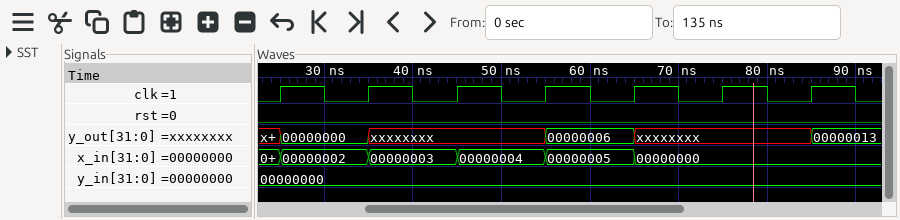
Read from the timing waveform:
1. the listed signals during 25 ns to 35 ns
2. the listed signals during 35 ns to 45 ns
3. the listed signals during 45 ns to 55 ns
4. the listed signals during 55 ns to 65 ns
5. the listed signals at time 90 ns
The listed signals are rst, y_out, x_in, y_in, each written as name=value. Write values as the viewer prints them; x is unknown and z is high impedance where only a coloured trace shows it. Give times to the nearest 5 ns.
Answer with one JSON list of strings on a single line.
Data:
["rst=0, y_out=00000000, x_in=00000002, y_in=00000000", "rst=0, y_out=xxxxxxxx, x_in=00000003, y_in=00000000", "rst=0, y_out=xxxxxxxx, x_in=00000004, y_in=00000000", "rst=0, y_out=00000006, x_in=00000005, y_in=00000000", "rst=0, y_out=00000013, x_in=00000000, y_in=00000000"]
